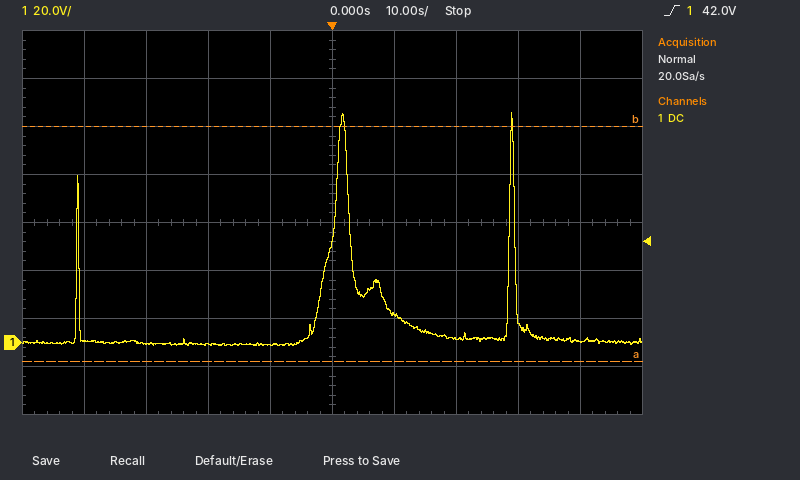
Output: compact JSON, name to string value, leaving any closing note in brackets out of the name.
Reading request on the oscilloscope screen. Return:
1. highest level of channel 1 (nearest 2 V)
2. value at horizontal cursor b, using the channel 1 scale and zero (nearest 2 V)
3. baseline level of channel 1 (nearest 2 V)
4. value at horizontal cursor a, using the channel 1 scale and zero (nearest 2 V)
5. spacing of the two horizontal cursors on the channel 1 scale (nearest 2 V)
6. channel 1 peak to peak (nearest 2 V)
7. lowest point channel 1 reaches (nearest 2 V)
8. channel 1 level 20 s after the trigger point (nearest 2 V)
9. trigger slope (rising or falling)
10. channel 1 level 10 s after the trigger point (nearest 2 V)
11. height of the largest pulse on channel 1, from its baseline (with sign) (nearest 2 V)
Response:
{"highest level of channel 1": "96 V", "value at horizontal cursor b, using the channel 1 scale and zero": "90 V", "baseline level of channel 1": "0 V", "value at horizontal cursor a, using the channel 1 scale and zero": "-8 V", "spacing of the two horizontal cursors on the channel 1 scale": "98 V", "channel 1 peak to peak": "98 V", "lowest point channel 1 reaches": "-2 V", "channel 1 level 20 s after the trigger point": "2 V", "trigger slope": "rising", "channel 1 level 10 s after the trigger point": "12 V", "height of the largest pulse on channel 1, from its baseline (with sign)": "+96 V"}
